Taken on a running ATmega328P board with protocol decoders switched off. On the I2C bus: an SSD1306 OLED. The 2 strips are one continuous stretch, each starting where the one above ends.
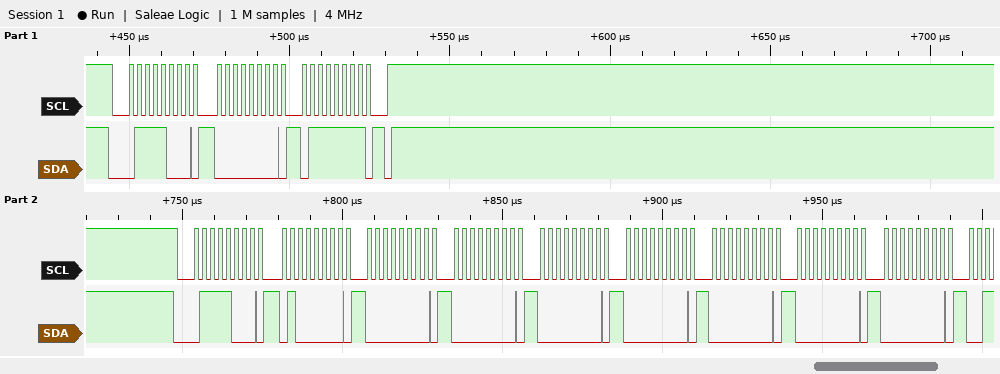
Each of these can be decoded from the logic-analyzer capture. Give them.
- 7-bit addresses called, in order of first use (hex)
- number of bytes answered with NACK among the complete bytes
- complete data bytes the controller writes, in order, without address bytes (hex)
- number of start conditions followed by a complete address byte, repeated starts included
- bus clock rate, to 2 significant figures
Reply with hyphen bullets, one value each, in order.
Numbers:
- 0x3C
- 0
- 00 7F 40 00 00 00 00 00 00 00
- 2
- 400 kHz
